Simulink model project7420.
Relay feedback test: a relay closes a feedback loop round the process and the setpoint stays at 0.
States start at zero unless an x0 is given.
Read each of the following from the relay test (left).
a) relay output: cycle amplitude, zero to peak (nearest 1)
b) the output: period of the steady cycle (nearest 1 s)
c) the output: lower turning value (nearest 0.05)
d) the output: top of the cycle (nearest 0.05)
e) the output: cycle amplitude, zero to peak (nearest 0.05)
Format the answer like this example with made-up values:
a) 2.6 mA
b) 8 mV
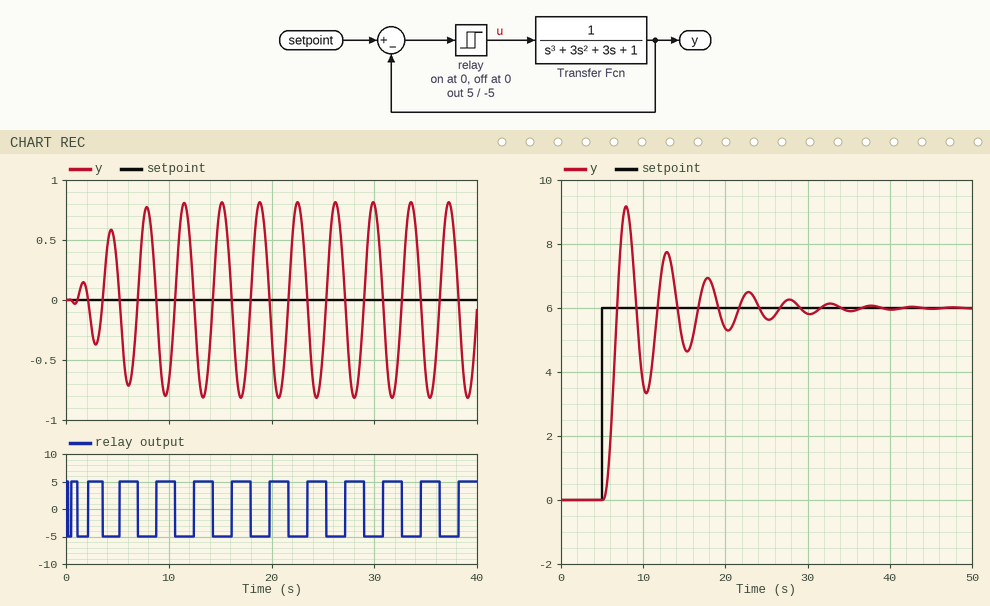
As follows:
a) 5
b) 4 s
c) -0.80
d) 0.80
e) 0.80
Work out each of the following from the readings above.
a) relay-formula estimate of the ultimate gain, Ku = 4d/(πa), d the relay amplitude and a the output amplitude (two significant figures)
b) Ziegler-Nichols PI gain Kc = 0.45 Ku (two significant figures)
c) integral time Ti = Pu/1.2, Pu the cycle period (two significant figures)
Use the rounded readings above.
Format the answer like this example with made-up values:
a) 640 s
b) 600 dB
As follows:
a) 8.0
b) 3.6
c) 3.3 s
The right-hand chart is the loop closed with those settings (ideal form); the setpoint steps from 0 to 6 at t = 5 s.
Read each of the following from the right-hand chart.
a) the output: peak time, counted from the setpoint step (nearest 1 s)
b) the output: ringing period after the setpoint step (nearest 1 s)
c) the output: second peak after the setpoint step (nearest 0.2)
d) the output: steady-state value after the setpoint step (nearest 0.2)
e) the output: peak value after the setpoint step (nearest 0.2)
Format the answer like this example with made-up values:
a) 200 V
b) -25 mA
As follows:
a) 3 s
b) 5 s
c) 7.8
d) 6.0
e) 9.2
